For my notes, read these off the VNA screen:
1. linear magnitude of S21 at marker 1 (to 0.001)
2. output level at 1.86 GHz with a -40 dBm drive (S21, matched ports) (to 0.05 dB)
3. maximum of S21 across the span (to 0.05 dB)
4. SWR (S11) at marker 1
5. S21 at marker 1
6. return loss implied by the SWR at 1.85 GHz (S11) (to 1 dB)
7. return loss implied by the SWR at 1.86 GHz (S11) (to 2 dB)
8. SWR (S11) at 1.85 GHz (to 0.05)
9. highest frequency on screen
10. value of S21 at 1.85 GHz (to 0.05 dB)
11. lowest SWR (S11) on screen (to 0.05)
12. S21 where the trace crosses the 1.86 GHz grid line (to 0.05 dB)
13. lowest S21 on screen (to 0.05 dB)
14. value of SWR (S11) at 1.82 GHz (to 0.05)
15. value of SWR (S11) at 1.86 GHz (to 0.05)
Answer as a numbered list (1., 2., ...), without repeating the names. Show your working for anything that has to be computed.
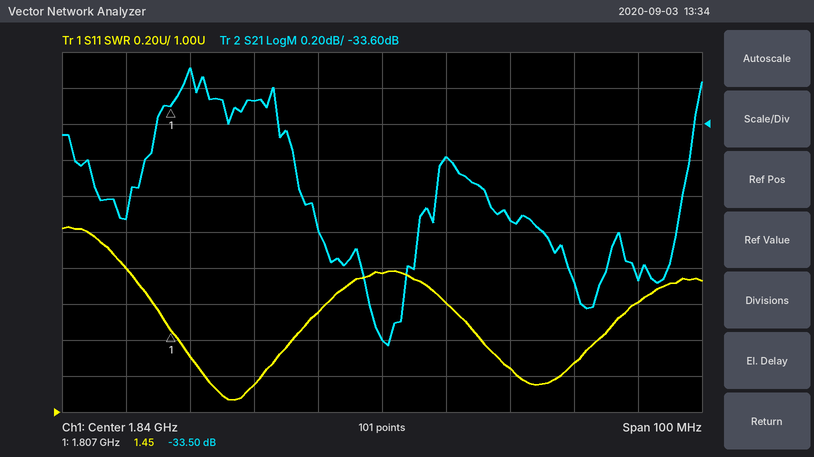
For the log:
1. 10^(-33.5/20) ≈ 0.021
2. -40 dBm + (-34.15 dB) = -74.15 dBm
3. -33.30 dB
4. 1.45
5. -33.50 dB
6. −20 log10((1.6 − 1)/(1.6 + 1)) ≈ 13 dB
7. −20 log10((1.25 − 1)/(1.25 + 1)) ≈ 19.1 dB, so 20 dB to the nearest 2 dB
8. 1.60
9. 1.89 GHz
10. -33.80 dB
11. 1.05
12. -34.15 dB
13. -34.85 dB
14. 1.15
15. 1.25
